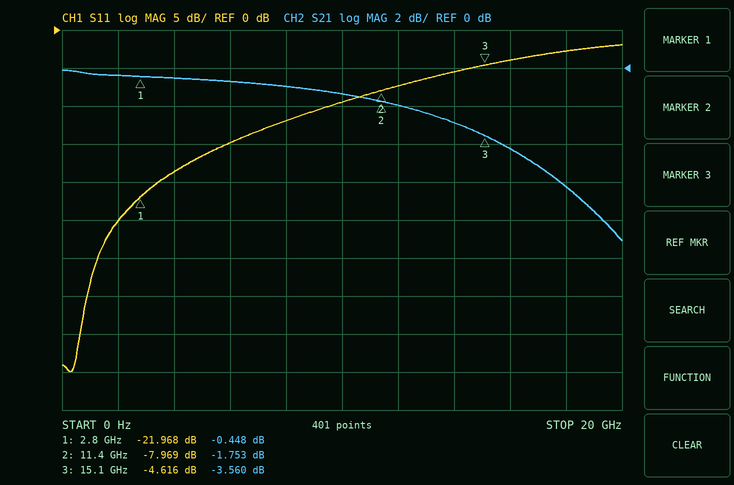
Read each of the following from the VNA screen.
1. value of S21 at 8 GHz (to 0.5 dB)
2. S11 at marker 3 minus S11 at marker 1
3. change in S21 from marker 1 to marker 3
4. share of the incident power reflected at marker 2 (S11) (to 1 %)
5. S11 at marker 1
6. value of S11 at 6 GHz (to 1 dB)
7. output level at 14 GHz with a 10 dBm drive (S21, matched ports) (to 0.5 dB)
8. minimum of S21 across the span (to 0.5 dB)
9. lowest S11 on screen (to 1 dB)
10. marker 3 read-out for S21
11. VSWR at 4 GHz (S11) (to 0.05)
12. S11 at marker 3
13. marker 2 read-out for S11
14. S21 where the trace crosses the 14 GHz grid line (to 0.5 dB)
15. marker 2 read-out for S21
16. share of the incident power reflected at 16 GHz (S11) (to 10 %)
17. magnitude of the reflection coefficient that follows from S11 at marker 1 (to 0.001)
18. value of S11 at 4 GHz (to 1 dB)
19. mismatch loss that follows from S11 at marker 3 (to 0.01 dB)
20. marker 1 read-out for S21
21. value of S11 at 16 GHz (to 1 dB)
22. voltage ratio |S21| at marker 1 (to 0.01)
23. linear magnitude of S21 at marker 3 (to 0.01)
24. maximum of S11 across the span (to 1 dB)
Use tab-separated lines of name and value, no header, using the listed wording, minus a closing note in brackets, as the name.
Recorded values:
value of S21 at 8 GHz	-1.0 dB
S11 at marker 3 minus S11 at marker 1	17.352 dB
change in S21 from marker 1 to marker 3	-3.112 dB
share of the incident power reflected at marker 2 (S11)	16 %
S11 at marker 1	-21.968 dB
value of S11 at 6 GHz	-15 dB
output level at 14 GHz with a 10 dBm drive (S21, matched ports)	7.0 dBm
minimum of S21 across the span	-9.0 dB
lowest S11 on screen	-45 dB
marker 3 read-out for S21	-3.560 dB
VSWR at 4 GHz (S11)	1.25
S11 at marker 3	-4.616 dB
marker 2 read-out for S11	-7.969 dB
S21 where the trace crosses the 14 GHz grid line	-3.0 dB
marker 2 read-out for S21	-1.753 dB
share of the incident power reflected at 16 GHz (S11)	40 %
magnitude of the reflection coefficient that follows from S11 at marker 1	0.080
value of S11 at 4 GHz	-19 dB
mismatch loss that follows from S11 at marker 3	1.84 dB
marker 1 read-out for S21	-0.448 dB
value of S11 at 16 GHz	-4 dB
voltage ratio |S21| at marker 1	0.95
linear magnitude of S21 at marker 3	0.66
maximum of S11 across the span	-2 dB
